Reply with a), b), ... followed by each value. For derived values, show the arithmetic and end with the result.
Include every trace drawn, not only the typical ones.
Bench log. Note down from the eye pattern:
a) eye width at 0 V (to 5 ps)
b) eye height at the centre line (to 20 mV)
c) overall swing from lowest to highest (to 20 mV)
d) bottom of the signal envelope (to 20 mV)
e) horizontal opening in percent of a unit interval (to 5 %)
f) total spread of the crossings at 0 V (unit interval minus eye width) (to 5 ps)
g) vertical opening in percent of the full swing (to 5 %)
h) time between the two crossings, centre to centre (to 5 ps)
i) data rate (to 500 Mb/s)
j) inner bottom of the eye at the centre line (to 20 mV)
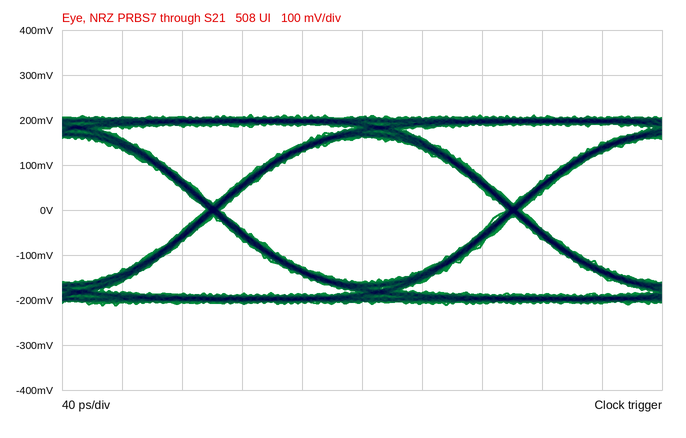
a) 190 ps
b) 320 mV
c) 420 mV
d) -220 mV
e) 190 ps / 200 ps ≈ 95 %
f) 10 ps
g) 320 mV / 420 mV ≈ 76.2 %, so 75 % to the nearest 5 %
h) 200 ps
i) 5.0 Gb/s
j) -160 mV
